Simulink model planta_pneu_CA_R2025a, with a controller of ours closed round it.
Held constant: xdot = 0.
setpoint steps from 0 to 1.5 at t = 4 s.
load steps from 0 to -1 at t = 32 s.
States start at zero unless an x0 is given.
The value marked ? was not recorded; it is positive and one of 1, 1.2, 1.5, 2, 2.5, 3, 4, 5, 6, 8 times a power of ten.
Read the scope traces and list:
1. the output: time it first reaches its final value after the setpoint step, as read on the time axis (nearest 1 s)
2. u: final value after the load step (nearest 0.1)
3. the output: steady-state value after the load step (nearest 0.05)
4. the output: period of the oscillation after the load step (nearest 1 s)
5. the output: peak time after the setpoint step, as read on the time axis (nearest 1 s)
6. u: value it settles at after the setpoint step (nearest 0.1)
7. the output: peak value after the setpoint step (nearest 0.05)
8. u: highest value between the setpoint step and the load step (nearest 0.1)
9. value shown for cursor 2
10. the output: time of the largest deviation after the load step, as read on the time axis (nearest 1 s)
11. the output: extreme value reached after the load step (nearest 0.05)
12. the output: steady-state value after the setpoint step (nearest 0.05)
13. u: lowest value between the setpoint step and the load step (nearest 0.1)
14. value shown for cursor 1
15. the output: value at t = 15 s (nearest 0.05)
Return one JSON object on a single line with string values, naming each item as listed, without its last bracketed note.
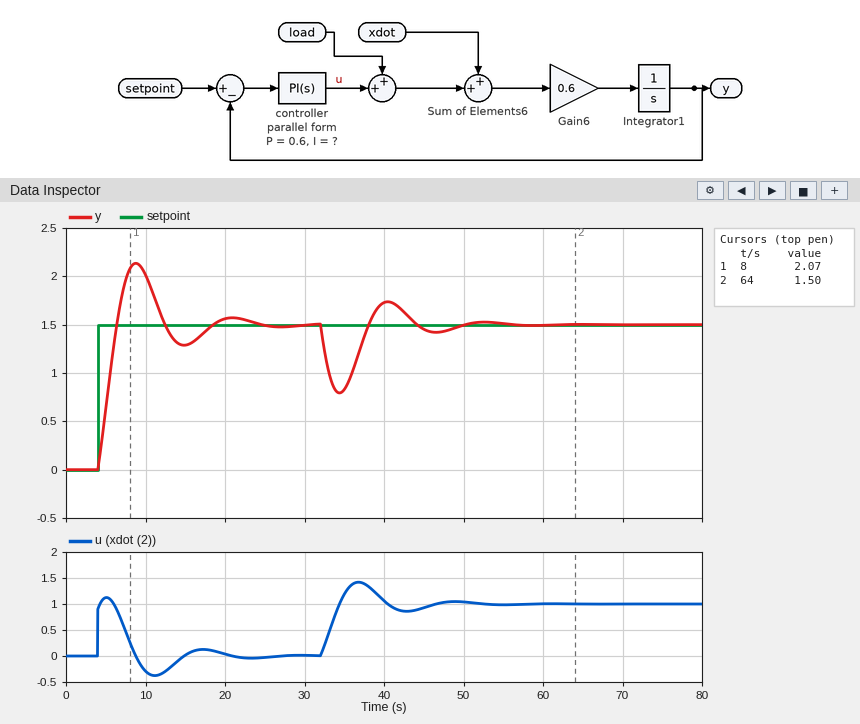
{"the output: time it first reaches its final value after the setpoint step, as read on the time axis": "6 s", "u: final value after the load step": "1.0", "the output: steady-state value after the load step": "1.50", "the output: period of the oscillation after the load step": "12 s", "the output: peak time after the setpoint step, as read on the time axis": "9 s", "u: value it settles at after the setpoint step": "0.0", "the output: peak value after the setpoint step": "2.15", "u: highest value between the setpoint step and the load step": "1.1", "value shown for cursor 2": "1.50", "the output: time of the largest deviation after the load step, as read on the time axis": "34 s", "the output: extreme value reached after the load step": "0.80", "the output: steady-state value after the setpoint step": "1.50", "u: lowest value between the setpoint step and the load step": "-0.4", "value shown for cursor 1": "2.07", "the output: value at t = 15 s": "1.30"}
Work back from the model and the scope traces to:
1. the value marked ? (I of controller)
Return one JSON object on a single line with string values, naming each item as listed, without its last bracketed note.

{"the value marked ?": "0.5"}
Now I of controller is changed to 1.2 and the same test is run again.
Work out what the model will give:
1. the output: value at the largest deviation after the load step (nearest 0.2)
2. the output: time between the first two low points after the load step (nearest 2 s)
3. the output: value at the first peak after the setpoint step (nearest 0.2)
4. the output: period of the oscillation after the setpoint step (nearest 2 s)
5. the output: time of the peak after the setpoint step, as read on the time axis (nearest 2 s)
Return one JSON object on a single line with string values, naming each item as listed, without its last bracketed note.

{"the output: value at the largest deviation after the load step": "1.0", "the output: time between the first two low points after the load step": "8 s", "the output: value at the first peak after the setpoint step": "2.4", "the output: period of the oscillation after the setpoint step": "8 s", "the output: time of the peak after the setpoint step, as read on the time axis": "8 s"}
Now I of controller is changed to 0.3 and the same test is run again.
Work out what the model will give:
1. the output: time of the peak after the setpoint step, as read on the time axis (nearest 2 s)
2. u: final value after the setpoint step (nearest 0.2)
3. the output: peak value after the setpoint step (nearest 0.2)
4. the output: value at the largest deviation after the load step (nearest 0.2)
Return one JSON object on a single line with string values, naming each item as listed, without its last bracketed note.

{"the output: time of the peak after the setpoint step, as read on the time axis": "10 s", "u: final value after the setpoint step": "0.0", "the output: peak value after the setpoint step": "2.0", "the output: value at the largest deviation after the load step": "0.6"}
